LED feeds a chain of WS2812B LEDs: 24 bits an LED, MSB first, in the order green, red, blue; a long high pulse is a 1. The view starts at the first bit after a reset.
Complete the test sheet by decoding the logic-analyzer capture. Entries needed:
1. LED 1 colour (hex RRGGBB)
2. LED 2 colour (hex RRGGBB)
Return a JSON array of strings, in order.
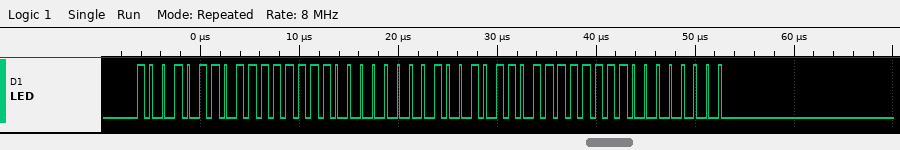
["#FF9600", "#FF9600"]
